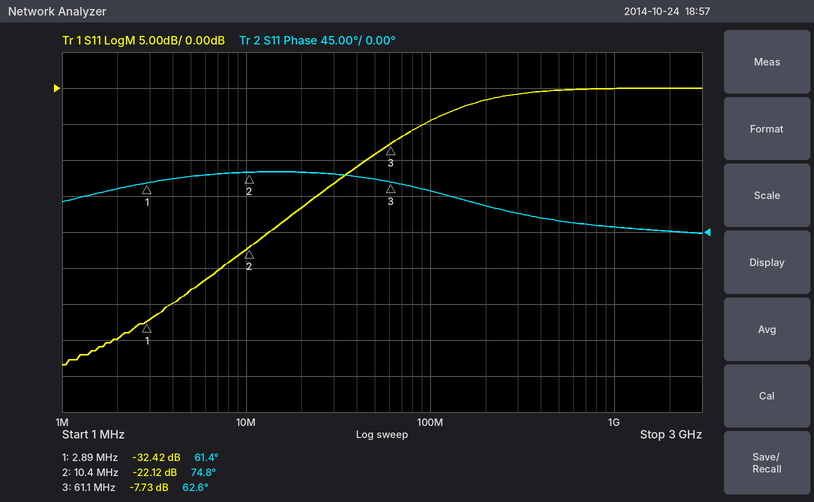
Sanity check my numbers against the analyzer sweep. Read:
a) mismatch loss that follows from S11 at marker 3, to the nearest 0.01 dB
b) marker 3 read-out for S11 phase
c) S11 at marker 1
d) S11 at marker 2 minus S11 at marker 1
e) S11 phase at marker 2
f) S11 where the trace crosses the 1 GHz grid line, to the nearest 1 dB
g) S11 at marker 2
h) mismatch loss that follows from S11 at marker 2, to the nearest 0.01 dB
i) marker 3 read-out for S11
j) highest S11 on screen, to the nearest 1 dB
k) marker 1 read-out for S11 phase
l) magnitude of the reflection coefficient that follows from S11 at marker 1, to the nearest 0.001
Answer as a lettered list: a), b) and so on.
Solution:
a) 0.80 dB
b) 62.6°
c) -32.42 dB
d) 10.30 dB
e) 74.8°
f) 0 dB
g) -22.12 dB
h) 0.03 dB
i) -7.73 dB
j) 0 dB
k) 61.4°
l) 0.024
